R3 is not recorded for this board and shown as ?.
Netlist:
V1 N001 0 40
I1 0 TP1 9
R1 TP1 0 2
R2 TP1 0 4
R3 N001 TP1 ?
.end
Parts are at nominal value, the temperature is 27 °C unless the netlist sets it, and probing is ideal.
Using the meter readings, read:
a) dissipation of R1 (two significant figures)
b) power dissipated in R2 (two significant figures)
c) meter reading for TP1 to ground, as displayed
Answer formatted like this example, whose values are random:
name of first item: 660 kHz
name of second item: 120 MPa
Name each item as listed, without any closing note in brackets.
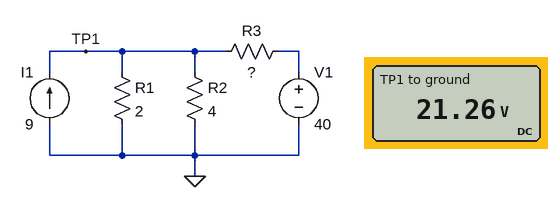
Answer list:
dissipation of R1: 230 W
power dissipated in R2: 110 W
meter reading for TP1 to ground, as displayed: 21.26 V
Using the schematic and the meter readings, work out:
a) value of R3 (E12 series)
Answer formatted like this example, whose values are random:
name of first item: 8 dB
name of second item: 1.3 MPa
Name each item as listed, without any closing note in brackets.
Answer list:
value of R3: 2.7 Ω
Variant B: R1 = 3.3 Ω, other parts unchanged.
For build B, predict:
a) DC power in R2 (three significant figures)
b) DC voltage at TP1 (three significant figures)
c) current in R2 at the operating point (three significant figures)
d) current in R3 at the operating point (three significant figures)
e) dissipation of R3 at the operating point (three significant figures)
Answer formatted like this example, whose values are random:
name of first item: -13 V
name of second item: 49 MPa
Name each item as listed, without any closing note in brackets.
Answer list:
DC power in R2: 166 W
DC voltage at TP1: 25.8 V
current in R2 at the operating point: 6.45 A
current in R3 at the operating point: 5.26 A
dissipation of R3 at the operating point: 74.8 W
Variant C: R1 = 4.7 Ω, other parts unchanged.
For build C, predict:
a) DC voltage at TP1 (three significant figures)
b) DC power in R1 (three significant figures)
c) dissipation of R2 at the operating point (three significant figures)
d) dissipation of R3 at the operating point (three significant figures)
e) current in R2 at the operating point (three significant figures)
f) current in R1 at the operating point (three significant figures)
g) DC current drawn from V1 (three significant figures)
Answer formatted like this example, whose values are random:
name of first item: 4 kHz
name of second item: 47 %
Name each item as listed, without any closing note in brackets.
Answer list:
DC voltage at TP1: 28.6 V
DC power in R1: 174 W
dissipation of R2 at the operating point: 204 W
dissipation of R3 at the operating point: 48.3 W
current in R2 at the operating point: 7.15 A
current in R1 at the operating point: 6.08 A
DC current drawn from V1: 4.23 A
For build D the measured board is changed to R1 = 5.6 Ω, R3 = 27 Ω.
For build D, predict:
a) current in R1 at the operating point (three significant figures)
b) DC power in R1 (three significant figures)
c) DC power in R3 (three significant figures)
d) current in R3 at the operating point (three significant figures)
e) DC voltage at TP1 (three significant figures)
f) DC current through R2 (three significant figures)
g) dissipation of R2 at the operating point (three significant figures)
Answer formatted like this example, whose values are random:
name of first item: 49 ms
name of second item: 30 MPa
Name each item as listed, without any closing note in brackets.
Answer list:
current in R1 at the operating point: 4.02 A
DC power in R1: 90.5 W
DC power in R3: 11.3 W
current in R3 at the operating point: 648 mA
DC voltage at TP1: 22.5 V
DC current through R2: 5.63 A
dissipation of R2 at the operating point: 127 W
